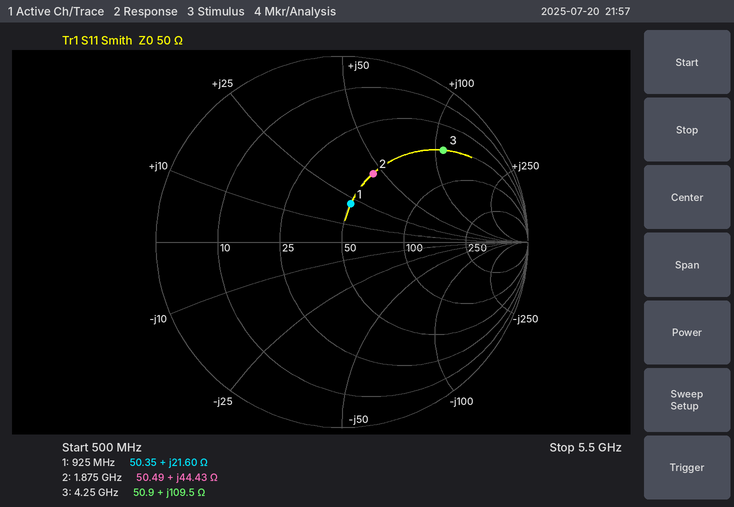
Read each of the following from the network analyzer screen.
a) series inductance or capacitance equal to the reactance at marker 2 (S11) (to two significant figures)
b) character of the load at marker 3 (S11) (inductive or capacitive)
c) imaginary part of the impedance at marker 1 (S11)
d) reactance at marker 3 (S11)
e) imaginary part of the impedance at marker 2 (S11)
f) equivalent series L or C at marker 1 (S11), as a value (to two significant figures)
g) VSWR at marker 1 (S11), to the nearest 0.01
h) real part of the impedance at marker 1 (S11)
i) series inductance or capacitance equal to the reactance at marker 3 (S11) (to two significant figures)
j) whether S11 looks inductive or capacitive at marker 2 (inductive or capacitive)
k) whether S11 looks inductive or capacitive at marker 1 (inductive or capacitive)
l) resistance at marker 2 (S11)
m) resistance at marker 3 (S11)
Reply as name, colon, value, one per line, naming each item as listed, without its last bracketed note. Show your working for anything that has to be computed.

series inductance or capacitance equal to the reactance at marker 2 (S11): L = 44.43 Ω/(2π × 1.875 GHz) ≈ 3.8 nH
character of the load at marker 3 (S11): inductive
imaginary part of the impedance at marker 1: +21.60 Ω
reactance at marker 3: +109.5 Ω
imaginary part of the impedance at marker 2: +44.43 Ω
equivalent series L or C at marker 1 (S11), as a value: L = 21.6 Ω/(2π × 925 MHz) ≈ 3.7 nH
VSWR at marker 1 (S11), to the nearest 0.01: 1.53
real part of the impedance at marker 1: 50.35 Ω
series inductance or capacitance equal to the reactance at marker 3 (S11): L = 109.5 Ω/(2π × 4.25 GHz) ≈ 4.1 nH
whether S11 looks inductive or capacitive at marker 2: inductive
whether S11 looks inductive or capacitive at marker 1: inductive
resistance at marker 2: 50.49 Ω
resistance at marker 3: 50.9 Ω
